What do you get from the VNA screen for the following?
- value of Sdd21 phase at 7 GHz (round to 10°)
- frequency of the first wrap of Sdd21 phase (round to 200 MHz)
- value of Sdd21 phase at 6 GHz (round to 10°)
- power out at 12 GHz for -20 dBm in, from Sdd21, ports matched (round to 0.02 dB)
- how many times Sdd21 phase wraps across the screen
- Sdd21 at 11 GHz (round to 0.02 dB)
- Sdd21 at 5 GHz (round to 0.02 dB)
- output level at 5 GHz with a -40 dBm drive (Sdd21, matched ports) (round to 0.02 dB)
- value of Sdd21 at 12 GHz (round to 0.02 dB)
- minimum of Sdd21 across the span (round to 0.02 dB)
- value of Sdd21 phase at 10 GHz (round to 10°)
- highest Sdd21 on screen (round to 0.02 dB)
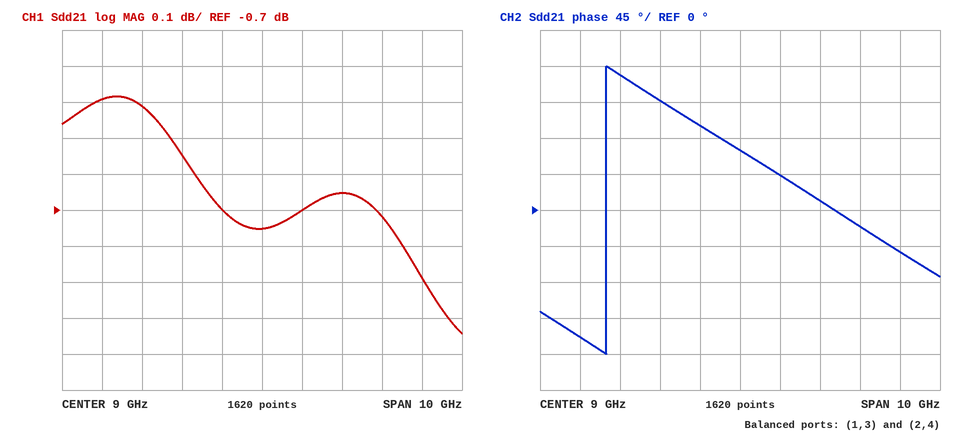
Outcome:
140°
5.6 GHz
170°
-20.72 dBm
1
-0.66 dB
-0.40 dB
-40.40 dBm
-0.72 dB
-1.04 dB
40°
-0.38 dB
